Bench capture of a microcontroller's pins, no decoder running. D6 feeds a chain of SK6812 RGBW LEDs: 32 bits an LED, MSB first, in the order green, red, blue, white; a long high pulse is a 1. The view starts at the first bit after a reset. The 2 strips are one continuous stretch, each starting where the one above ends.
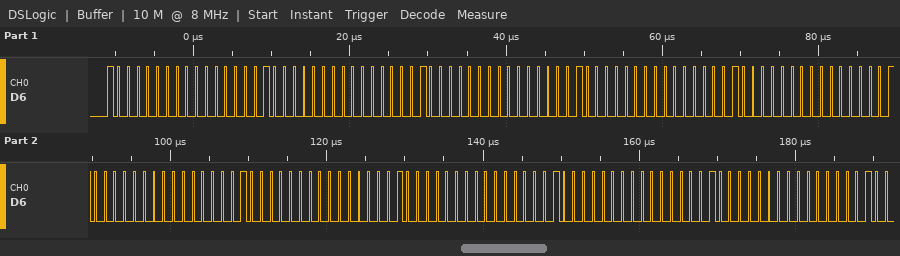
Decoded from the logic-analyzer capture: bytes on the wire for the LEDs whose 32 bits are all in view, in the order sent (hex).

80 00 80 00 80 00 80 00 80 00 80 00 80 00 80 00 80 00 80 00
